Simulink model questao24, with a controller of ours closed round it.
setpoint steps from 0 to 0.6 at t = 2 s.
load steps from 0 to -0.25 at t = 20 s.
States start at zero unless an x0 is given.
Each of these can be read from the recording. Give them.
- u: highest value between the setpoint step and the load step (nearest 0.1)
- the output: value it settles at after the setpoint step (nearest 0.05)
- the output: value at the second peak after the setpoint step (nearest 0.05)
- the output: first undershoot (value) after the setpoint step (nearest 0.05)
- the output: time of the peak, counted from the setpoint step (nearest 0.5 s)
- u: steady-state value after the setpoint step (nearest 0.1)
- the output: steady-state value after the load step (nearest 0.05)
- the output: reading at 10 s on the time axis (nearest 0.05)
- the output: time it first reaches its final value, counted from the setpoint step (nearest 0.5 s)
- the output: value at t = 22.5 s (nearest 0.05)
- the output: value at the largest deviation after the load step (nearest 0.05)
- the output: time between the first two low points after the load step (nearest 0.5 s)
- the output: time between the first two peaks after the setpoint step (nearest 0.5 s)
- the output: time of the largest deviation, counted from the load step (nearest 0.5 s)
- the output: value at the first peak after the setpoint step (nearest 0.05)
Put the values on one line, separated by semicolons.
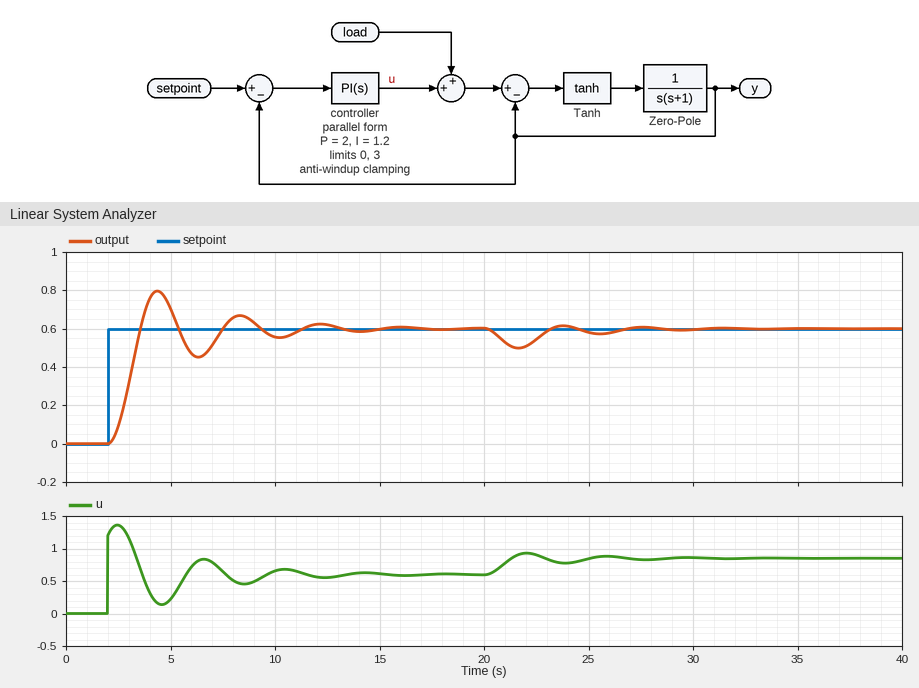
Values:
1.4; 0.60; 0.65; 0.45; 2.5 s; 0.6; 0.60; 0.55; 1.5 s; 0.55; 0.50; 4.0 s; 4.0 s; 1.5 s; 0.80
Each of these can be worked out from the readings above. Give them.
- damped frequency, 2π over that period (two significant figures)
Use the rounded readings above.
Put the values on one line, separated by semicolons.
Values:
1.6 rad/s
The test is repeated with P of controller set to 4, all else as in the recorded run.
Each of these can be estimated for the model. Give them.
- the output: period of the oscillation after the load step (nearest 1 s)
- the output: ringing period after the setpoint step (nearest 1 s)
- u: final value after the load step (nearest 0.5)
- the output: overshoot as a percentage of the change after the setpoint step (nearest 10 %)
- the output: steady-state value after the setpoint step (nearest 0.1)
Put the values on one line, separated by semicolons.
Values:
3 s; 3 s; 1.0; 30 %; 0.6
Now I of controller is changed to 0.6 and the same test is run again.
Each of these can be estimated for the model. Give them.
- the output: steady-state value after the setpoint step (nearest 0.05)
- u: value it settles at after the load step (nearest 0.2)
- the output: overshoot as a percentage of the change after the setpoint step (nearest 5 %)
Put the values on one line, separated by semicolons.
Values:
0.60; 0.8; 10 %
